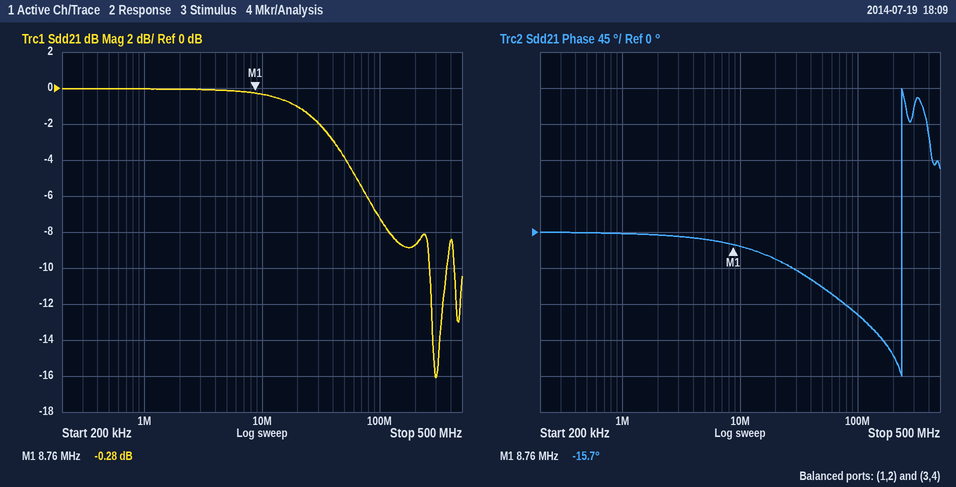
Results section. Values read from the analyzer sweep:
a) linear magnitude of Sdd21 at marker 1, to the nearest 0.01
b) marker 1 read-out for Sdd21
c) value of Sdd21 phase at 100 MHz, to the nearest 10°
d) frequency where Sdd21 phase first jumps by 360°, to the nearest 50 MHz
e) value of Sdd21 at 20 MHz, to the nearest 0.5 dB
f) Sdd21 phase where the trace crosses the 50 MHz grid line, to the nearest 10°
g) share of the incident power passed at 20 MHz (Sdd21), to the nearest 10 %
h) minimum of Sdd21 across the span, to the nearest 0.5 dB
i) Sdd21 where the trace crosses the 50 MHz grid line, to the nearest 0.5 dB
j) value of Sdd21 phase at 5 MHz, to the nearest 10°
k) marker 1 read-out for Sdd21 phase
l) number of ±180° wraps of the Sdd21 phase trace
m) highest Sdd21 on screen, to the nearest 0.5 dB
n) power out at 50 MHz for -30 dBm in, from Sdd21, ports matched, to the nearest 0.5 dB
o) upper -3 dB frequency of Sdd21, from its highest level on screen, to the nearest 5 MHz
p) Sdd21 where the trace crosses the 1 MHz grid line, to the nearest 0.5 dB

0.97
-0.28 dB
-100°
250 MHz
-1.0 dB
-70°
80 %
-16.0 dB
-4.0 dB
-10°
-15.7°
1
0.0 dB
-34.0 dBm
40 MHz
0.0 dB
